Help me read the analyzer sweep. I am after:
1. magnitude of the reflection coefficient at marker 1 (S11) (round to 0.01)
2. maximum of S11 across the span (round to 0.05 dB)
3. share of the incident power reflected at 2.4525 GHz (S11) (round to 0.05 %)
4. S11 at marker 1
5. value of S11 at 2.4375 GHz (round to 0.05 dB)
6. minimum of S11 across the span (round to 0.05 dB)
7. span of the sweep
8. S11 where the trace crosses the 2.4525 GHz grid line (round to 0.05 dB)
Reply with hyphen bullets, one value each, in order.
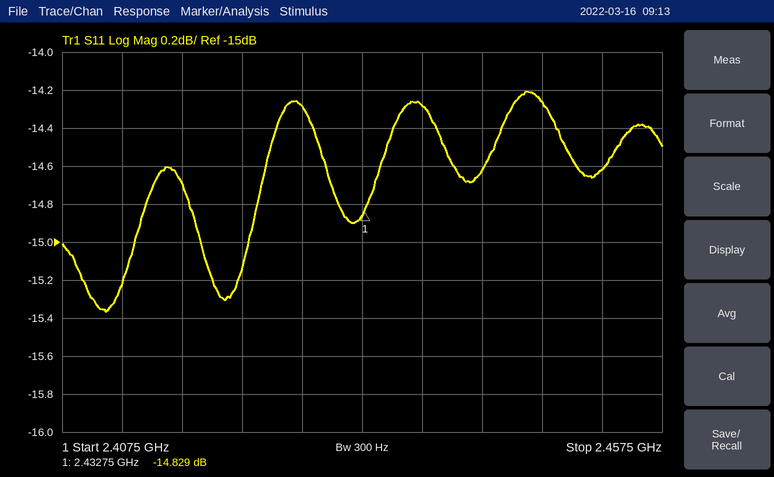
- 0.18
- -14.20 dB
- 3.45 %
- -14.829 dB
- -14.30 dB
- -15.35 dB
- 50 MHz
- -14.60 dB
